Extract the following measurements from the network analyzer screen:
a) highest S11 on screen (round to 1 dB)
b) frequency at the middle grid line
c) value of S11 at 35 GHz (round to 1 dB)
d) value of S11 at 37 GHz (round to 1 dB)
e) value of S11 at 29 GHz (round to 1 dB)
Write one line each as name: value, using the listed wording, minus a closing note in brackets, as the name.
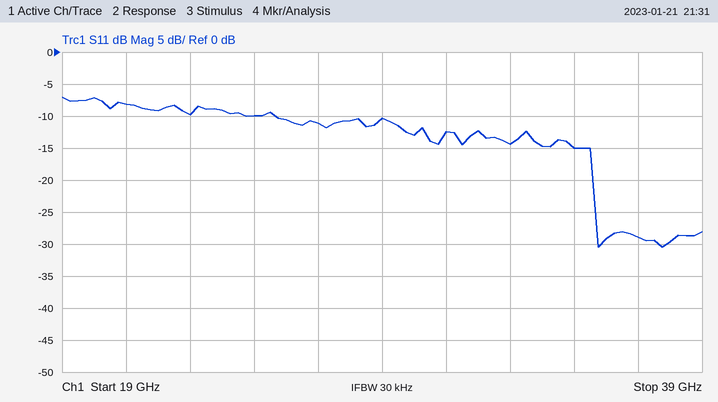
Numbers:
highest S11 on screen: -7 dB
frequency at the middle grid line: 29 GHz
value of S11 at 35 GHz: -15 dB
value of S11 at 37 GHz: -29 dB
value of S11 at 29 GHz: -10 dB
